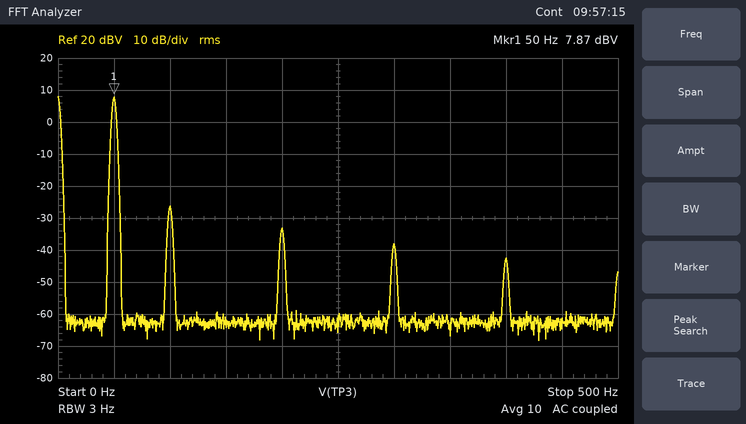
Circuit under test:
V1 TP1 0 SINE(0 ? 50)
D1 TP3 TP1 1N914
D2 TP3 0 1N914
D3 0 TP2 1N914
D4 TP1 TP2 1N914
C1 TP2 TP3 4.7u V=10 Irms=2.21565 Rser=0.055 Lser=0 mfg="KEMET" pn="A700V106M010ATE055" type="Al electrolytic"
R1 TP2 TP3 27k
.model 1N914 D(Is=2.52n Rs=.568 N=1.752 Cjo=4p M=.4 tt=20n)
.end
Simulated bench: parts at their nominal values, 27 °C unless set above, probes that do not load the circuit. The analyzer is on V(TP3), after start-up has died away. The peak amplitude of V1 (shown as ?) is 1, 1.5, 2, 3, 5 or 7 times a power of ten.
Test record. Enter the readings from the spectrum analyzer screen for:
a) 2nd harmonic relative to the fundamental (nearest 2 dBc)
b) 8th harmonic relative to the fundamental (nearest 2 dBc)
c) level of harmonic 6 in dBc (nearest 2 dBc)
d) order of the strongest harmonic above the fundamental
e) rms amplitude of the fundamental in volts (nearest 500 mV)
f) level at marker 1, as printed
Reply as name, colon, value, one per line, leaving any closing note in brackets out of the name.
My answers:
2nd harmonic relative to the fundamental: -34 dBc
8th harmonic relative to the fundamental: -50 dBc
level of harmonic 6 in dBc: -46 dBc
order of the strongest harmonic above the fundamental: 2
rms amplitude of the fundamental in volts: 2.5 V
level at marker 1, as printed: 7.87 dBV
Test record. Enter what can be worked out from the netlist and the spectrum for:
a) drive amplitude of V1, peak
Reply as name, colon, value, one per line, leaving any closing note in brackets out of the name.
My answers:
drive amplitude of V1, peak: 7 V
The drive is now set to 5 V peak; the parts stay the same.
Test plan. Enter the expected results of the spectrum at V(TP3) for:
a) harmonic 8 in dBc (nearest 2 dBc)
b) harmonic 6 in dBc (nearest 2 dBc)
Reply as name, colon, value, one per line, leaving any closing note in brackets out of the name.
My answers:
harmonic 8 in dBc: -52 dBc
harmonic 6 in dBc: -48 dBc
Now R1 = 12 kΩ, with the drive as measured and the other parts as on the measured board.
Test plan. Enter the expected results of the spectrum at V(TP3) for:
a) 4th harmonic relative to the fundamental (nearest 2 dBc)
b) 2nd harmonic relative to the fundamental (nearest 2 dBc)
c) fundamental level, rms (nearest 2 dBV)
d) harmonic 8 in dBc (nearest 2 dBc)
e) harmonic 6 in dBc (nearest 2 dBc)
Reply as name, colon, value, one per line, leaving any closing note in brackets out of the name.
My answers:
4th harmonic relative to the fundamental: -34 dBc
2nd harmonic relative to the fundamental: -28 dBc
fundamental level, rms: 8 dBV
harmonic 8 in dBc: -46 dBc
harmonic 6 in dBc: -40 dBc
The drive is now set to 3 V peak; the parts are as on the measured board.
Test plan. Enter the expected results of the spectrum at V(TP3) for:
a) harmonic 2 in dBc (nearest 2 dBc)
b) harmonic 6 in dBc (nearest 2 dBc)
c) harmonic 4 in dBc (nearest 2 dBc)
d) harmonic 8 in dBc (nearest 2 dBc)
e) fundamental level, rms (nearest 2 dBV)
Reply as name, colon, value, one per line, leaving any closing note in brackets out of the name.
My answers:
harmonic 2 in dBc: -36 dBc
harmonic 6 in dBc: -50 dBc
harmonic 4 in dBc: -44 dBc
harmonic 8 in dBc: -56 dBc
fundamental level, rms: 0 dBV
